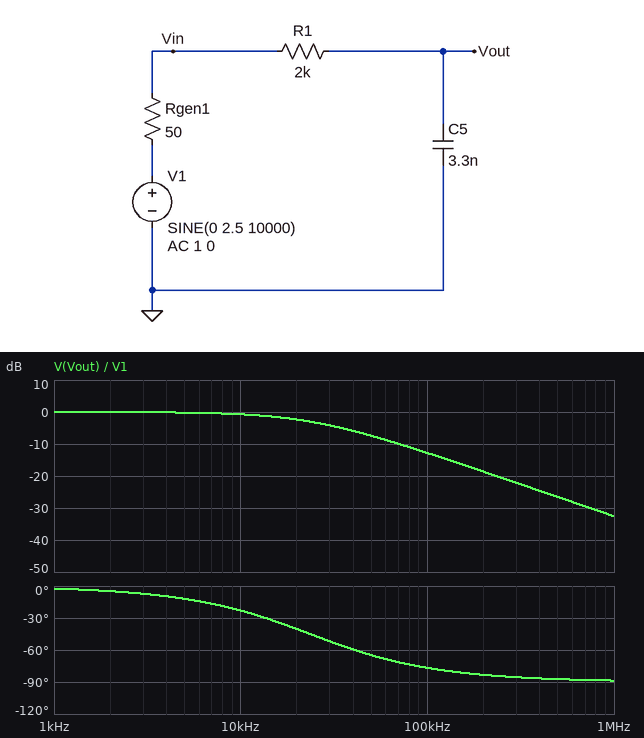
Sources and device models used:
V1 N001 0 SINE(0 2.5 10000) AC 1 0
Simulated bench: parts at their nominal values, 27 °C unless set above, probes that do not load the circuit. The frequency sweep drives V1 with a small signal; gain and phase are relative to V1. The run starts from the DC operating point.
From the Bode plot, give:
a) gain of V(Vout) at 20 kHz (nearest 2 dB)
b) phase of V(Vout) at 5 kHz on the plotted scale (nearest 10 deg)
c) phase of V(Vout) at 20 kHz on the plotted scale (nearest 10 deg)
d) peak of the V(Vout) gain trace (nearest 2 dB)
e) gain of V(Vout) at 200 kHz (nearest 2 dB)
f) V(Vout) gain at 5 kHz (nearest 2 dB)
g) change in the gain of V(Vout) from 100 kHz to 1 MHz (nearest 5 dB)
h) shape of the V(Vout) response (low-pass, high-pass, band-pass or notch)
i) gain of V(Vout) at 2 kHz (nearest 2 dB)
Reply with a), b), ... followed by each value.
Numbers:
a) -2 dB
b) -10 deg
c) -40 deg
d) 0 dB
e) -18 dB
f) 0 dB
g) -20 dB
h) low-pass
i) 0 dB
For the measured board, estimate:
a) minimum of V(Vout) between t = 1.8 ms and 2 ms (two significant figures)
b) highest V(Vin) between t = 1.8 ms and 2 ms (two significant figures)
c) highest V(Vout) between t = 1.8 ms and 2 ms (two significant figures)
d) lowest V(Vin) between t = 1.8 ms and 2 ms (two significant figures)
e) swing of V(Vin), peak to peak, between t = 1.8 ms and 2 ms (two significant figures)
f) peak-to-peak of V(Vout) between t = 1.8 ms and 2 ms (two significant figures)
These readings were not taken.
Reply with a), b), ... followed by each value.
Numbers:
a) -2.3 V
b) 2.5 V
c) 2.3 V
d) -2.5 V
e) 5.0 V
f) 4.6 V
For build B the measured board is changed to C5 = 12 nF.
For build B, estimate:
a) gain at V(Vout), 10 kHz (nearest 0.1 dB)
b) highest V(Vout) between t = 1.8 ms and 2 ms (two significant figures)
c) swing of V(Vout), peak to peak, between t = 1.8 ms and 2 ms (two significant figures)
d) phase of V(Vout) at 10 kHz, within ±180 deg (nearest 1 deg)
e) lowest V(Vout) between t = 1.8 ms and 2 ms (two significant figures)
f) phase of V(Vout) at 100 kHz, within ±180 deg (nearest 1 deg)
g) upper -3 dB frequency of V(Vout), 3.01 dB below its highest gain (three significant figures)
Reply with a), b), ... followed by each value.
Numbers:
a) -5.3 dB
b) 1.4 V
c) 2.7 V
d) -57 deg
e) -1.4 V
f) -86 deg
g) 6.47 kHz
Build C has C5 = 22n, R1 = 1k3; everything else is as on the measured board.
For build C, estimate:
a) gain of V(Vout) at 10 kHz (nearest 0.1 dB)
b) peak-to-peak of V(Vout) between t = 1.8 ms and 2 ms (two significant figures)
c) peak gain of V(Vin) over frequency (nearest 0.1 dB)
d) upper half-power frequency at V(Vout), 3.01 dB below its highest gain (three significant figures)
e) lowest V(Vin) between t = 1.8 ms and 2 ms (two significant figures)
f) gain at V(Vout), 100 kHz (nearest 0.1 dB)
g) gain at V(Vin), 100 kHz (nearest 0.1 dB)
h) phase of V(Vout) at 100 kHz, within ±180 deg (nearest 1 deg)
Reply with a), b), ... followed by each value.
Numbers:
a) -6.5 dB
b) 2.4 V
c) 0 dB
d) 5.36 kHz
e) -2.4 V
f) -25.4 dB
g) -0.3 dB
h) -87 deg
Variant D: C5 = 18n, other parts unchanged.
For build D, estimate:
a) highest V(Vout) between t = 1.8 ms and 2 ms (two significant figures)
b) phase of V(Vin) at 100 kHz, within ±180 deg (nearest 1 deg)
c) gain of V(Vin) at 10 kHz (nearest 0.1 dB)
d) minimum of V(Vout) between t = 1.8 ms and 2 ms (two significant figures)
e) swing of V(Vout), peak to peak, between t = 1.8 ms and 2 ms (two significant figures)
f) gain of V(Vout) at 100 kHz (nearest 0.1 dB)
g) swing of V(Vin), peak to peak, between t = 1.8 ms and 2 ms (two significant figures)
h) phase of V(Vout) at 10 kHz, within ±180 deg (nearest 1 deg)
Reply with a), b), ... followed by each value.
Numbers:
a) 990 mV
b) 0 deg
c) -0.2 dB
d) -990 mV
e) 2.0 V
f) -27.3 dB
g) 4.9 V
h) -67 deg
